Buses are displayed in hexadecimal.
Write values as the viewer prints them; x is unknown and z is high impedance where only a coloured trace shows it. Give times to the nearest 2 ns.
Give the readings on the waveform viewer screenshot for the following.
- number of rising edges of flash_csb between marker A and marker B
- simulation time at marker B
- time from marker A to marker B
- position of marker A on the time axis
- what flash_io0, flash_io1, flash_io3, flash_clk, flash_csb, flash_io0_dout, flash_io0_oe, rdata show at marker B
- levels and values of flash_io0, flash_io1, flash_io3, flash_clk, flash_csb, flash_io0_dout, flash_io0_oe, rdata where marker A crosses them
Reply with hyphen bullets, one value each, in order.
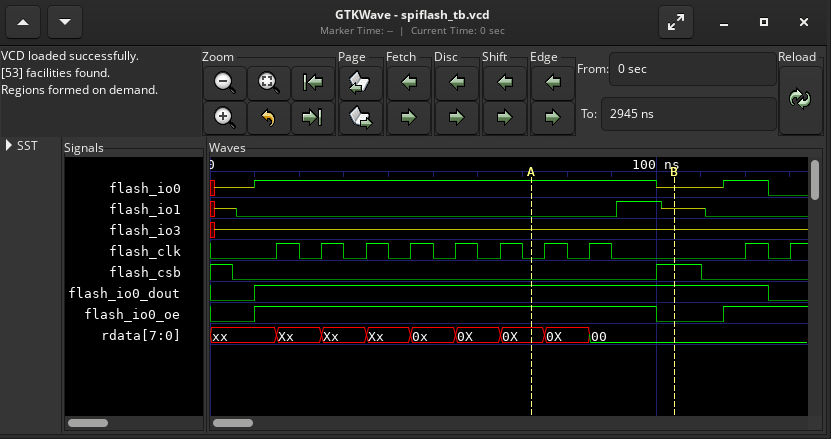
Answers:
- 1
- 104 ns
- 32 ns
- 72 ns
- flash_io0=z, flash_io1=z, flash_io3=z, flash_clk=0, flash_csb=1, flash_io0_dout=1, flash_io0_oe=0, rdata=00
- flash_io0=1, flash_io1=0, flash_io3=z, flash_clk=0, flash_csb=0, flash_io0_dout=1, flash_io0_oe=1, rdata=0X
